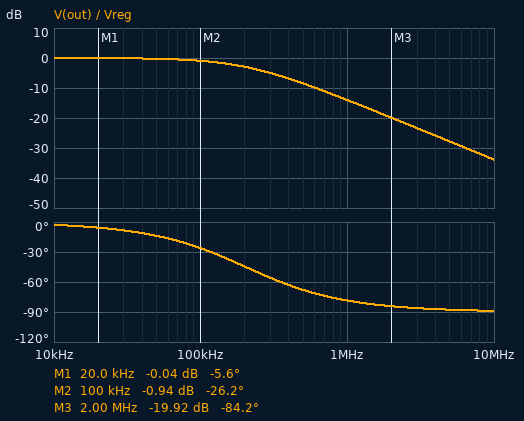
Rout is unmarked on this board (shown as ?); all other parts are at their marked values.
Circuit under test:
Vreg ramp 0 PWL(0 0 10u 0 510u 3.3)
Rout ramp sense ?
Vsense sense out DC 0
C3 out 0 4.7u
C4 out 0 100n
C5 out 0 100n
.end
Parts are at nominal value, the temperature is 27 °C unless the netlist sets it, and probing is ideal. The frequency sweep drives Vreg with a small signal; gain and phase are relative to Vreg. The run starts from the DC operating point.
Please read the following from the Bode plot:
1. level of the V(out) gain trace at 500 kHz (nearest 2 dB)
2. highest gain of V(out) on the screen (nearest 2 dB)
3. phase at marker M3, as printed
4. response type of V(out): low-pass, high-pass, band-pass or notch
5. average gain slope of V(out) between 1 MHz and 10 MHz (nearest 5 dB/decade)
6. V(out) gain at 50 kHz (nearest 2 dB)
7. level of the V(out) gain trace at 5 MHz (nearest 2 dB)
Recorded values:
-8 dB
0 dB
-84.2 deg
low-pass
-20 dB/decade
0 dB
-28 dB
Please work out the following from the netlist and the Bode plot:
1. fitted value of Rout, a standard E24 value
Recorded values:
0.16 Ω
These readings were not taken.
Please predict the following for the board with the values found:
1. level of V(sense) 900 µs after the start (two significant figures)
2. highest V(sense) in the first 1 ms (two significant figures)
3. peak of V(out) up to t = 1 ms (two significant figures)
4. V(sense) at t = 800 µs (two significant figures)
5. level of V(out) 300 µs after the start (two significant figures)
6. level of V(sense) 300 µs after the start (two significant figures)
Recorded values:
3.3 V
3.3 V
3.3 V
3.3 V
1.9 V
1.9 V
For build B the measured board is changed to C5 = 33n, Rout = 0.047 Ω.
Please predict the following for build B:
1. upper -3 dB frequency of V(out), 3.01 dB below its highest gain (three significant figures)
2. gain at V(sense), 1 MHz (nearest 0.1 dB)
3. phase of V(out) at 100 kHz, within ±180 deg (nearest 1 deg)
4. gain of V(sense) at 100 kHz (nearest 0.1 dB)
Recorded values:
701 kHz
-4.8 dB
-8 deg
-0.1 dB
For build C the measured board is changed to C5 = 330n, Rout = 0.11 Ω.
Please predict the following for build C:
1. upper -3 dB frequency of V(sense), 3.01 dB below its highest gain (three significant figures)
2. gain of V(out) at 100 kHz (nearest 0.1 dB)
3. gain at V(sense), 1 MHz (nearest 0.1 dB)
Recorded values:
282 kHz
-0.5 dB
-11.3 dB
